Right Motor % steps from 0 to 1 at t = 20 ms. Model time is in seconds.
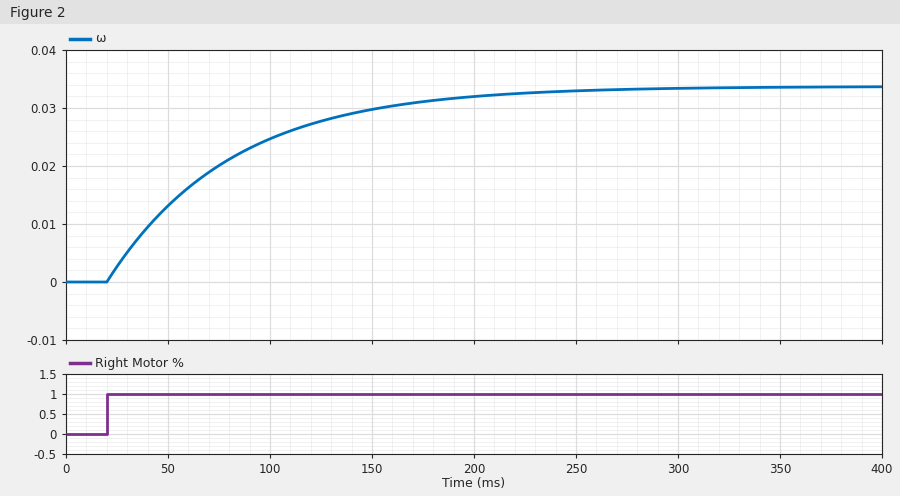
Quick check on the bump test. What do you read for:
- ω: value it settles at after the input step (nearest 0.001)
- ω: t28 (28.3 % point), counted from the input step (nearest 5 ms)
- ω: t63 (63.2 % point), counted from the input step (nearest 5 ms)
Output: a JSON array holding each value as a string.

["0.034", "20 ms", "60 ms"]
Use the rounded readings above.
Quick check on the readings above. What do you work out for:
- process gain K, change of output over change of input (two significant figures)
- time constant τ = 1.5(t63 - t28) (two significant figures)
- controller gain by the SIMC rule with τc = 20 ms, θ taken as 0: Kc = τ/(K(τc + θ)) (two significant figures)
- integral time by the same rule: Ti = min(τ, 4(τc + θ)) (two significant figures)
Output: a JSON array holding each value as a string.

["0.034", "60 ms", "88", "60 ms"]
